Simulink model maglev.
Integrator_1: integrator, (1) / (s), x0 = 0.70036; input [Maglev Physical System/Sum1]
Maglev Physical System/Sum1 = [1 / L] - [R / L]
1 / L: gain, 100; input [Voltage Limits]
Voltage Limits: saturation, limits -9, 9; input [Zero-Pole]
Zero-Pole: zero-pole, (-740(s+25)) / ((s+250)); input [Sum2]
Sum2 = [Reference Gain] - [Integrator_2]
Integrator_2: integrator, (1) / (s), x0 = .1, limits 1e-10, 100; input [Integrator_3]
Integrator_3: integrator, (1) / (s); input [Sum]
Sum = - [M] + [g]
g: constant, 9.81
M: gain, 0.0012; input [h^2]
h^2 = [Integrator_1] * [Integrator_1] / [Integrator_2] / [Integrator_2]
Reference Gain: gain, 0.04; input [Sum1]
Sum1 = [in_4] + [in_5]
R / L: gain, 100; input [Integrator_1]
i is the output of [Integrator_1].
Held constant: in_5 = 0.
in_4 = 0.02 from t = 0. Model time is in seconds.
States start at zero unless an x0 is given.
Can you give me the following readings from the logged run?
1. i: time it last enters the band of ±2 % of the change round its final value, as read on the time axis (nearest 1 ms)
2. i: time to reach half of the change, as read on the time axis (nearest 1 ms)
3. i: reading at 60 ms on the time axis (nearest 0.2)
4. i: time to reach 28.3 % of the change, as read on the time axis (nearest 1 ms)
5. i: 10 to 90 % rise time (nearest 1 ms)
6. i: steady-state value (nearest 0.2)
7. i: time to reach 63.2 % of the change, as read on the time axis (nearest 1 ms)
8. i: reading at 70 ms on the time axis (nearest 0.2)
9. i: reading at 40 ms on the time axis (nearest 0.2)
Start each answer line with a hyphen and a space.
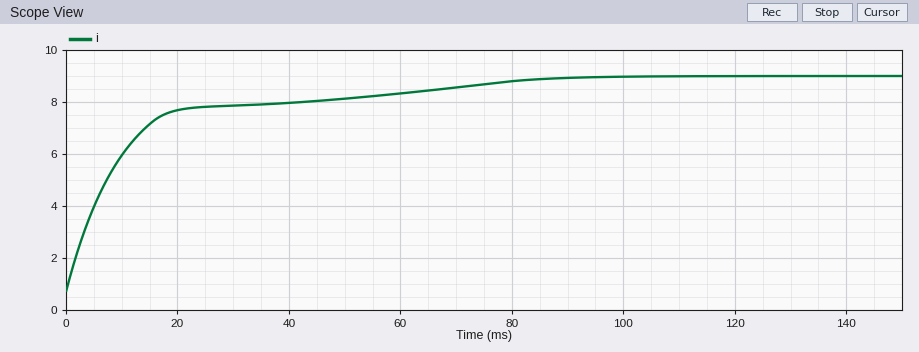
- 82 ms
- 7 ms
- 8.4
- 3 ms
- 51 ms
- 9.0
- 10 ms
- 8.6
- 8.0
